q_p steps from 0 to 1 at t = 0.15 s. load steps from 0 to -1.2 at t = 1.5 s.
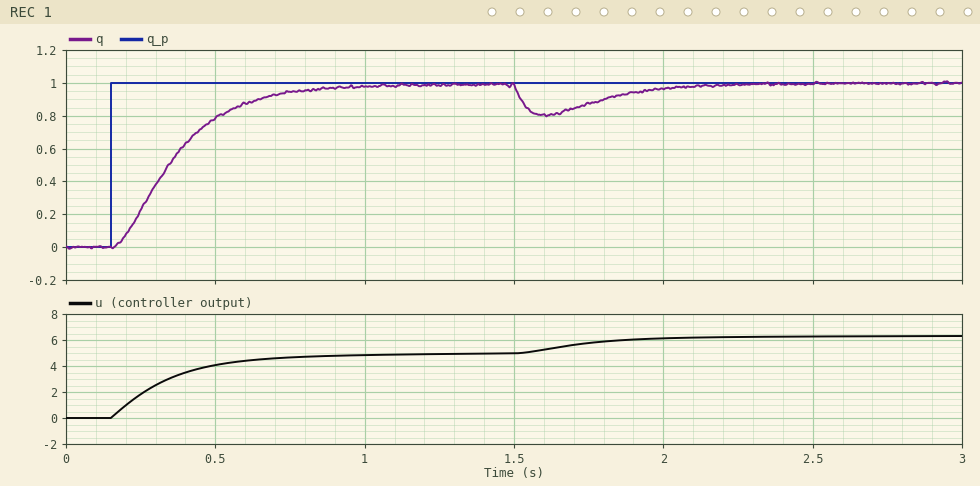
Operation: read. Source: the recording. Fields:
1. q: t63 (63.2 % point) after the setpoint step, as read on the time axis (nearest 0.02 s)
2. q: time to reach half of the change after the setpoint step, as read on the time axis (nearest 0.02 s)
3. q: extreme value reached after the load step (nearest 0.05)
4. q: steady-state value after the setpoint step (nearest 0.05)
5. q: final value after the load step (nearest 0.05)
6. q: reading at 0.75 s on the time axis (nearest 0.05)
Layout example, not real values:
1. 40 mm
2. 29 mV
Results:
1. 0.40 s
2. 0.34 s
3. 0.80
4. 1.00
5. 1.00
6. 0.95
